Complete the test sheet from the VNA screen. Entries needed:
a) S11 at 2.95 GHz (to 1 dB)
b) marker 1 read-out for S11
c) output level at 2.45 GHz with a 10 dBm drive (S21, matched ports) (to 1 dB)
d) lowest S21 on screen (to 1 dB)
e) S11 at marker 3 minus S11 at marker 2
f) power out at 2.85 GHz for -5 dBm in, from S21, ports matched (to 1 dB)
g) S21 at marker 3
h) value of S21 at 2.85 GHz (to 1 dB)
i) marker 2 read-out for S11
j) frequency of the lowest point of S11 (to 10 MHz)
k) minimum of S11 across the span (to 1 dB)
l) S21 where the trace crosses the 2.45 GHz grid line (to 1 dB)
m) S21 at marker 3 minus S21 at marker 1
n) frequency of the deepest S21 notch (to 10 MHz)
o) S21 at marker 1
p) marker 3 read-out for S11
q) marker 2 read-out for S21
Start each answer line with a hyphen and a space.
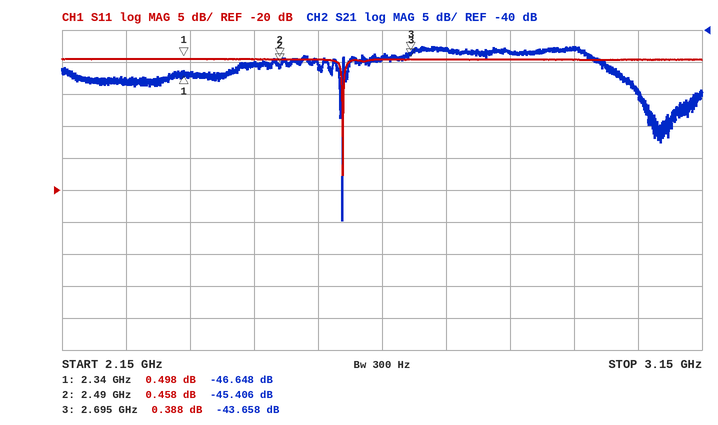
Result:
- 0 dB
- 0.498 dB
- -35 dBm
- -70 dB
- -0.070 dB
- -49 dBm
- -43.658 dB
- -44 dB
- 0.458 dB
- 2.59 GHz
- -18 dB
- -45 dB
- 2.990 dB
- 2.59 GHz
- -46.648 dB
- 0.388 dB
- -45.406 dB
